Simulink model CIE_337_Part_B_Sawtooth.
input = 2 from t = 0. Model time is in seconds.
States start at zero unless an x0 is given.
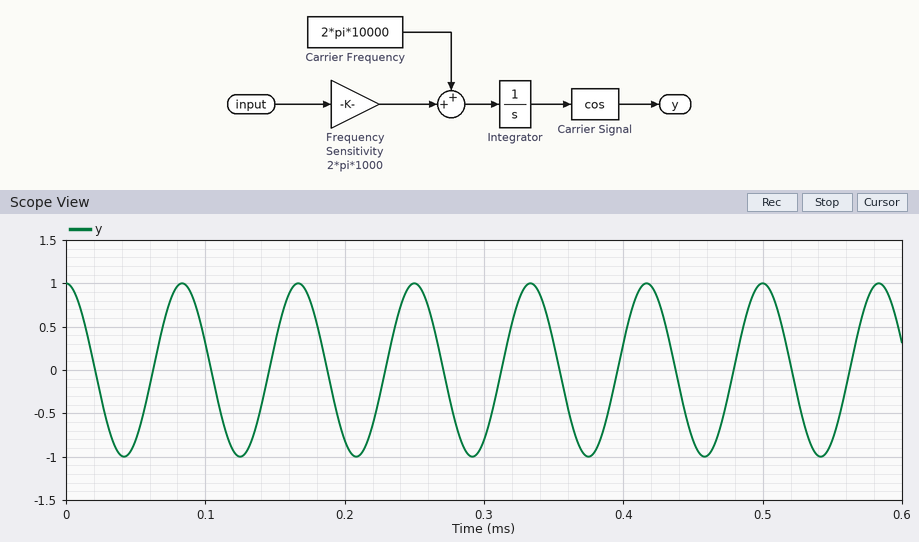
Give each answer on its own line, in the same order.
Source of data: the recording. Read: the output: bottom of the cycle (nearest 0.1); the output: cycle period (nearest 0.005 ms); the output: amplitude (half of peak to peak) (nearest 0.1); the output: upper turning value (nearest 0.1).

-1.0
0.085 ms
1.0
1.0
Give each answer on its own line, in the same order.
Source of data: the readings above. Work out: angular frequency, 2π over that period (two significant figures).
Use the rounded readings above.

74 rad/ms
